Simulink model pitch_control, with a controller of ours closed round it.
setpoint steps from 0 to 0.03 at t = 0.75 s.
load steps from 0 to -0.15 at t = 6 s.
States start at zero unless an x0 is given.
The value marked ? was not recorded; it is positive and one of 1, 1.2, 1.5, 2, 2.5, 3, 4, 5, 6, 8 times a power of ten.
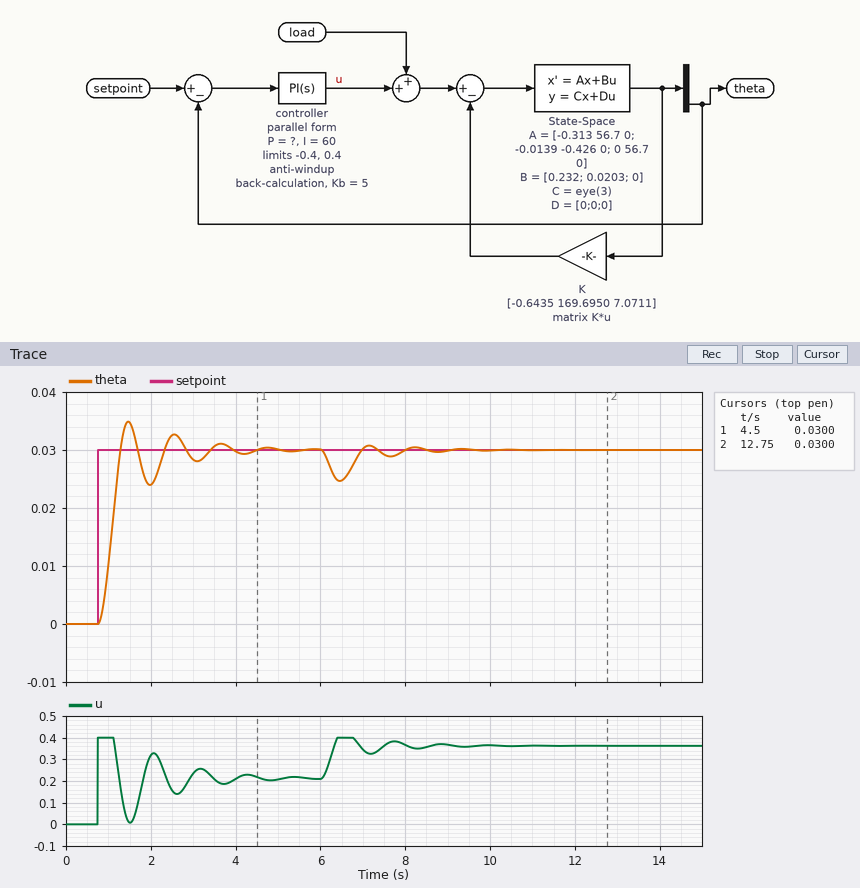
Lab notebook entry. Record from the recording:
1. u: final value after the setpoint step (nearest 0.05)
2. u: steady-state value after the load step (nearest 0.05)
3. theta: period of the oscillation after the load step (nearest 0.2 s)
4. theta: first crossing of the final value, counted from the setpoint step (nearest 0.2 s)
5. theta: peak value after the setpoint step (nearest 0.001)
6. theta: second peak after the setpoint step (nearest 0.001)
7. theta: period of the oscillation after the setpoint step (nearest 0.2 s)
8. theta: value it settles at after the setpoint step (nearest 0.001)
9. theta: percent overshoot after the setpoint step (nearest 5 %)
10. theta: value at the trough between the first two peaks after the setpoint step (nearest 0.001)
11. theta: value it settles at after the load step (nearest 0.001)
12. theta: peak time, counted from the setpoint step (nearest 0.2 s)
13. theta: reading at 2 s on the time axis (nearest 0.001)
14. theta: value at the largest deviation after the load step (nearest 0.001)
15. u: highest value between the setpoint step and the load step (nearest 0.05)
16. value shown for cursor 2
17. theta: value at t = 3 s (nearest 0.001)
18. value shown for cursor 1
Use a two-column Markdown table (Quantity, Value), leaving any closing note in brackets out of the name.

| Quantity | Value |
|---|---|
| u: final value after the setpoint step | 0.20 |
| u: steady-state value after the load step | 0.35 |
| theta: period of the oscillation after the load step | 1.2 s |
| theta: first crossing of the final value, counted from the setpoint step | 0.6 s |
| theta: peak value after the setpoint step | 0.035 |
| theta: second peak after the setpoint step | 0.033 |
| theta: period of the oscillation after the setpoint step | 1.0 s |
| theta: value it settles at after the setpoint step | 0.030 |
| theta: percent overshoot after the setpoint step | 15 % |
| theta: value at the trough between the first two peaks after the setpoint step | 0.024 |
| theta: value it settles at after the load step | 0.030 |
| theta: peak time, counted from the setpoint step | 0.8 s |
| theta: reading at 2 s on the time axis | 0.024 |
| theta: value at the largest deviation after the load step | 0.025 |
| u: highest value between the setpoint step and the load step | 0.40 |
| value shown for cursor 2 | 0.0300 |
| theta: value at t = 3 s | 0.028 |
| value shown for cursor 1 | 0.0300 |
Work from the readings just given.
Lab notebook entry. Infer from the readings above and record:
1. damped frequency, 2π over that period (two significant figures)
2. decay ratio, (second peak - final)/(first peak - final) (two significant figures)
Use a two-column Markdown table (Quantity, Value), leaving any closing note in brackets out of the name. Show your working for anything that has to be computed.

| Quantity | Value |
|---|---|
| damped frequency, 2π over that period | 2π / 1 = 6.3 rad/s |
| decay ratio, (second peak - final)/(first peak - final) | (0.033 - 0.03) / (0.035 - 0.03) = 0.60 |
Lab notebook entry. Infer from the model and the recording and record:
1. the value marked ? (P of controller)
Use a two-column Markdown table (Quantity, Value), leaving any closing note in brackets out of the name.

| Quantity | Value |
|---|---|
| the value marked ? | 25 |
